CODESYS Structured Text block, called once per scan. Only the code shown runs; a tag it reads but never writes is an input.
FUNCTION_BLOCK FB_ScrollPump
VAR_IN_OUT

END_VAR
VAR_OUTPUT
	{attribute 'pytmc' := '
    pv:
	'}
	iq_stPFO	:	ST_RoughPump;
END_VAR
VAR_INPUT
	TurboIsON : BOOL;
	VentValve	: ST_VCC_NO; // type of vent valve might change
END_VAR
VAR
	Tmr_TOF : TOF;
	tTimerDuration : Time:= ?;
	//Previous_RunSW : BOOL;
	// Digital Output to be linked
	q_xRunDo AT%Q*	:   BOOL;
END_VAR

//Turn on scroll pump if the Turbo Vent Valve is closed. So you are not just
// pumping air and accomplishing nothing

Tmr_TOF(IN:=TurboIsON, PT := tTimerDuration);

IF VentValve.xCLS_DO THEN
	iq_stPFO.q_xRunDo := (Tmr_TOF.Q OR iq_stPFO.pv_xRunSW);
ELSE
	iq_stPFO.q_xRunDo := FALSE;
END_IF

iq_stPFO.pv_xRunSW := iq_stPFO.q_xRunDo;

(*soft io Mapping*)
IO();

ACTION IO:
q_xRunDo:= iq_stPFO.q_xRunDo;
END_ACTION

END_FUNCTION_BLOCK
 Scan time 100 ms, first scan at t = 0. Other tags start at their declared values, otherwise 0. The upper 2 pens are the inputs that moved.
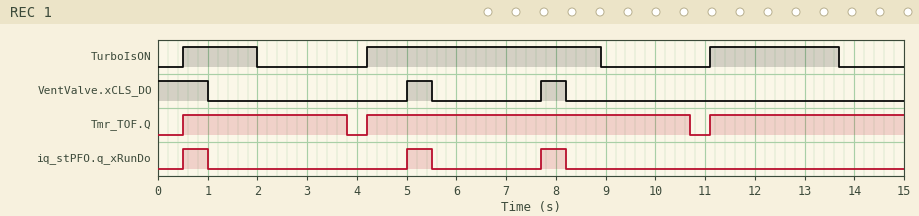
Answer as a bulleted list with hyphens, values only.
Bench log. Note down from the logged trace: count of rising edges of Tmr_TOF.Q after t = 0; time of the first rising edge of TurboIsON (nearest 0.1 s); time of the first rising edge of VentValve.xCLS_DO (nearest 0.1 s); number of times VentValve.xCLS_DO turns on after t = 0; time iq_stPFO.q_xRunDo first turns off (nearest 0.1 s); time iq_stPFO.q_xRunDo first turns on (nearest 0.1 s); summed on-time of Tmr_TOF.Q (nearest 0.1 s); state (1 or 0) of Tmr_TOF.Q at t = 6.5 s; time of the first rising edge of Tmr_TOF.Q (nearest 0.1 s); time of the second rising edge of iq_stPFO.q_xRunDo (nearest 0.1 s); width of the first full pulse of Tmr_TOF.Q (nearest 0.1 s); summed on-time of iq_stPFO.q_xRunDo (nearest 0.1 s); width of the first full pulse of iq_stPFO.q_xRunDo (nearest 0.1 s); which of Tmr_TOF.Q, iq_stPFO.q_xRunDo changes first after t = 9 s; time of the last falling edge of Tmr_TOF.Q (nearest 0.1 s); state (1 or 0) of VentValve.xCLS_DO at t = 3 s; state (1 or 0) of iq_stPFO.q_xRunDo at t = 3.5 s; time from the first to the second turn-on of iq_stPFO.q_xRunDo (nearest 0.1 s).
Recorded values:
- 3
- 0.5 s
- 5.0 s
- 2
- 1.0 s
- 0.5 s
- 13.7 s
- 1
- 0.5 s
- 5.0 s
- 3.3 s
- 1.5 s
- 0.5 s
- Tmr_TOF.Q
- 10.7 s
- 0
- 0
- 4.5 s
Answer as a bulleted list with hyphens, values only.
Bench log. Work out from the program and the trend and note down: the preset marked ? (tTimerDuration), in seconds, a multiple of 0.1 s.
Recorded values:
- 1.8 s
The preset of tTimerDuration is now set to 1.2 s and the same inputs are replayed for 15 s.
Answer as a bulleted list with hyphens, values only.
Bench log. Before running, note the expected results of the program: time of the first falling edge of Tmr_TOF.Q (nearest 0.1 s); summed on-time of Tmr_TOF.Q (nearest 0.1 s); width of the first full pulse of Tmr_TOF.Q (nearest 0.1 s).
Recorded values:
- 3.2 s
- 12.4 s
- 2.7 s
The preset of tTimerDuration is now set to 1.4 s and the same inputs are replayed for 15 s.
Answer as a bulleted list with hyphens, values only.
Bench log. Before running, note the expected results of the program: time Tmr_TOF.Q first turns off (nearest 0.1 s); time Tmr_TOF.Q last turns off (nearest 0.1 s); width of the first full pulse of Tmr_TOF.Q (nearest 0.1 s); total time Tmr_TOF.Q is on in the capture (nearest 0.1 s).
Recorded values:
- 3.4 s
- 10.3 s
- 2.9 s
- 12.9 s
